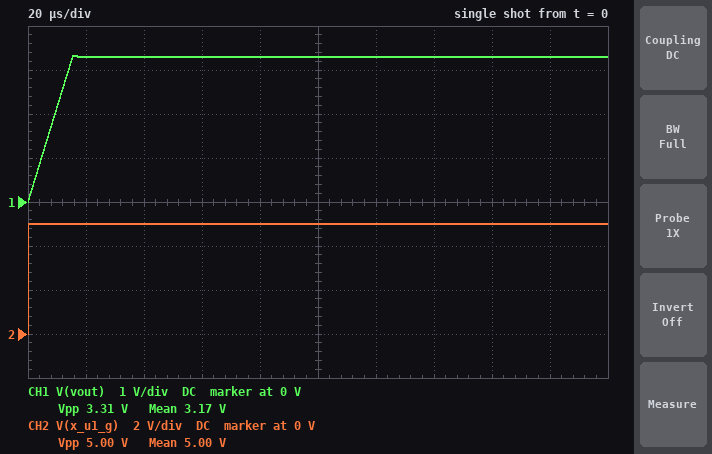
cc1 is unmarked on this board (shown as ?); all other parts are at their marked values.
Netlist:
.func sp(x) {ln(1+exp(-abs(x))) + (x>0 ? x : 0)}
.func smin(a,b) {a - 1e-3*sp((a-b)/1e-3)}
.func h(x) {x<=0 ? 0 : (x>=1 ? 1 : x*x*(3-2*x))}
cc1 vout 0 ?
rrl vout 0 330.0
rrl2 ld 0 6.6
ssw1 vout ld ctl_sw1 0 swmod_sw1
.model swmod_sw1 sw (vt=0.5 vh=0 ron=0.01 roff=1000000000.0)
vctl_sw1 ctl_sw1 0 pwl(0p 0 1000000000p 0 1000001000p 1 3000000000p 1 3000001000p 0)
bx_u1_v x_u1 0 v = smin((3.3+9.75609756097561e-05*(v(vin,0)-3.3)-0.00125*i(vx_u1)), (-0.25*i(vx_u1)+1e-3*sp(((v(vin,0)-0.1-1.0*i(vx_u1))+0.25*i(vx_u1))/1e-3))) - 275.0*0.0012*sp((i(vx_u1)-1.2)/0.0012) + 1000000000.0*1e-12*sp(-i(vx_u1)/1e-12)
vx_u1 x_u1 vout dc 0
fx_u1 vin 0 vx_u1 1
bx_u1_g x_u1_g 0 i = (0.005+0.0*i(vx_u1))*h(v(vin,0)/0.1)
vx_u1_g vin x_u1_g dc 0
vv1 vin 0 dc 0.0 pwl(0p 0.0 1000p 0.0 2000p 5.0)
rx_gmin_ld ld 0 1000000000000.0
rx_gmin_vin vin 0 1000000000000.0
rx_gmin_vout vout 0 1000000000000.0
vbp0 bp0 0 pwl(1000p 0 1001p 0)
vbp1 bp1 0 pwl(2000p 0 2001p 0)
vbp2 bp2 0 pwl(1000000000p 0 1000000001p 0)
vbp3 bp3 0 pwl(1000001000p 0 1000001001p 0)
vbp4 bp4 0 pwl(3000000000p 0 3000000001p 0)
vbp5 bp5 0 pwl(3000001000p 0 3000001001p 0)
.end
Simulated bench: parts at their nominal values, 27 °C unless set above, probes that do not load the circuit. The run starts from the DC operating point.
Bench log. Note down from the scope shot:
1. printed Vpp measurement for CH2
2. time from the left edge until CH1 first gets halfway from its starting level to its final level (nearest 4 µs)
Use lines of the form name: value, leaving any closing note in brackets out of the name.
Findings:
printed Vpp measurement for CH2: 5.00 V
time from the left edge until CH1 first gets halfway from its starting level to its final level: 8 µs
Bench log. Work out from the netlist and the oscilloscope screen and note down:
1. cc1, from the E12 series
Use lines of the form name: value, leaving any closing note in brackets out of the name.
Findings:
cc1, from the E12 series: 5.6 µF
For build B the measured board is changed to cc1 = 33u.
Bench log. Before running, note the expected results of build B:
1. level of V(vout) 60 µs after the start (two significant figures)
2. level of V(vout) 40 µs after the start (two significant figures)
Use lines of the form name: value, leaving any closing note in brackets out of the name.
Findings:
level of V(vout) 60 µs after the start: 2.2 V
level of V(vout) 40 µs after the start: 1.5 V
